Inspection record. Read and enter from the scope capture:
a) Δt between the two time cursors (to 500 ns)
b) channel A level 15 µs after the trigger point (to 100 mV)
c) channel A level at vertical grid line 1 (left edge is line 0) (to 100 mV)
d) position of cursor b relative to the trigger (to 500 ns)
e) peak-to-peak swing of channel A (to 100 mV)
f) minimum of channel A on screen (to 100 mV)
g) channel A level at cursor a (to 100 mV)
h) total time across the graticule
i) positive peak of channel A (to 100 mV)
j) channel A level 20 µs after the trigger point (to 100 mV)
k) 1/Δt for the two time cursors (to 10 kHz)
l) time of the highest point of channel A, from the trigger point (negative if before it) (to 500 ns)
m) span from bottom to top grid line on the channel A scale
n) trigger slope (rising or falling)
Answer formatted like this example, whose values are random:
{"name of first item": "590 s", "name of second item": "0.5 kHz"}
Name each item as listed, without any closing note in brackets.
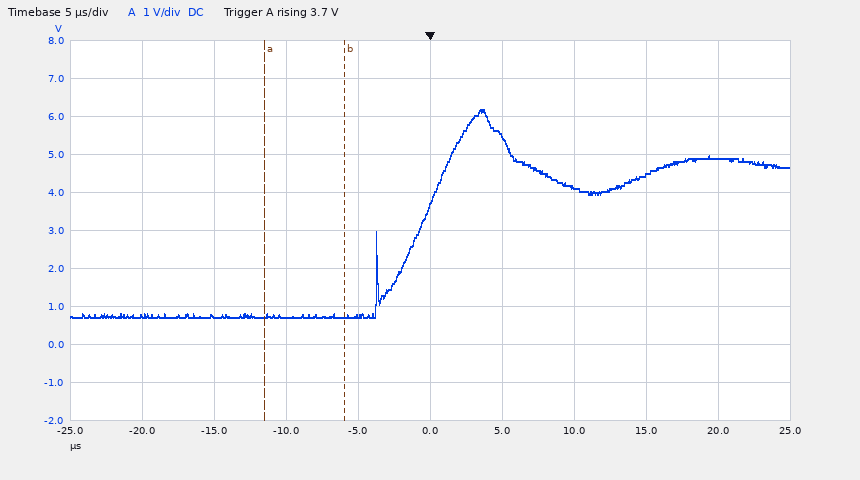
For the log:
{"Δt between the two time cursors": "5.5 µs", "channel A level 15 µs after the trigger point": "4.5 V", "channel A level at vertical grid line 1 (left edge is line 0)": "800 mV", "position of cursor b relative to the trigger": "-6.0 µs", "peak-to-peak swing of channel A": "5.5 V", "minimum of channel A on screen": "700 mV", "channel A level at cursor a": "800 mV", "total time across the graticule": "50 µs", "positive peak of channel A": "6.2 V", "channel A level 20 µs after the trigger point": "4.9 V", "1/Δt for the two time cursors": "180 kHz", "time of the highest point of channel A, from the trigger point (negative if before it)": "+3.5 µs", "span from bottom to top grid line on the channel A scale": "10 V", "trigger slope": "rising"}
